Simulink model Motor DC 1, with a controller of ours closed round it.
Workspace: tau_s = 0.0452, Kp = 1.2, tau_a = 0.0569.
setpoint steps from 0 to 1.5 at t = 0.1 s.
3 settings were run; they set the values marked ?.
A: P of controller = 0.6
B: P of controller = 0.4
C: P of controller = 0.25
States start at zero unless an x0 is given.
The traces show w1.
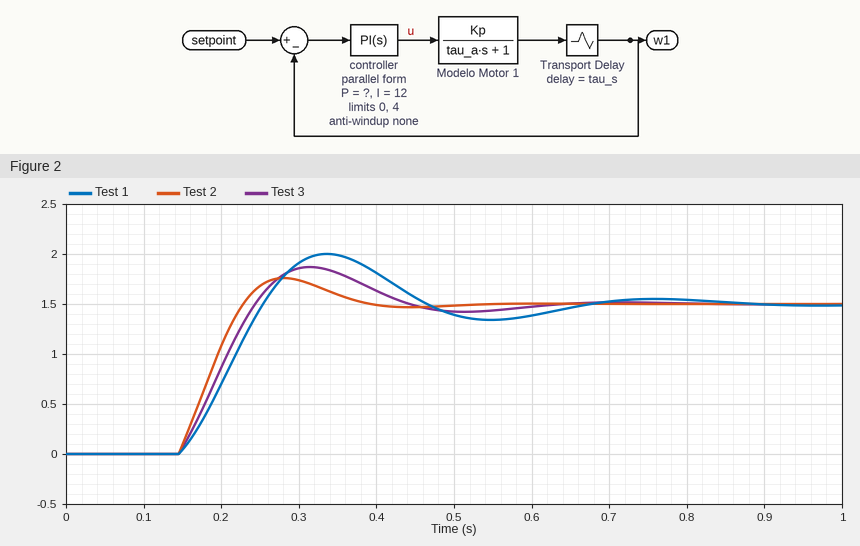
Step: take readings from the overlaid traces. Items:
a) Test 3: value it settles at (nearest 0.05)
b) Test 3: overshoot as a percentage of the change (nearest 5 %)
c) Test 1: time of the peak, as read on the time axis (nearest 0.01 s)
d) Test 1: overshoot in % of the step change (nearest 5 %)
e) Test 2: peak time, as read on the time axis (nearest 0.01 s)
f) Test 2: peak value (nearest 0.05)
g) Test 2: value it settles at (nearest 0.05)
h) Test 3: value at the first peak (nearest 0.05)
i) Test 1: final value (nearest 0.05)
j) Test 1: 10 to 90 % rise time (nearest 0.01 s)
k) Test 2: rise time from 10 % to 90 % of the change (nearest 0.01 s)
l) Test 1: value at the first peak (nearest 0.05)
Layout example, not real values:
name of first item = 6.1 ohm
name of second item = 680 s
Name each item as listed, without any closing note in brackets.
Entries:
Test 3: value it settles at = 1.50
Test 3: overshoot as a percentage of the change = 25 %
Test 1: time of the peak, as read on the time axis = 0.34 s
Test 1: overshoot in % of the step change = 35 %
Test 2: peak time, as read on the time axis = 0.28 s
Test 2: peak value = 1.75
Test 2: value it settles at = 1.50
Test 3: value at the first peak = 1.85
Test 1: final value = 1.50
Test 1: 10 to 90 % rise time = 0.08 s
Test 2: rise time from 10 % to 90 % of the change = 0.06 s
Test 1: value at the first peak = 2.00
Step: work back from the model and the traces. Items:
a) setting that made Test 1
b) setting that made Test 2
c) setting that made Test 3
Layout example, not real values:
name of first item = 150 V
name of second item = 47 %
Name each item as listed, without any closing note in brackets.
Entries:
setting that made Test 1 = C
setting that made Test 2 = A
setting that made Test 3 = B
